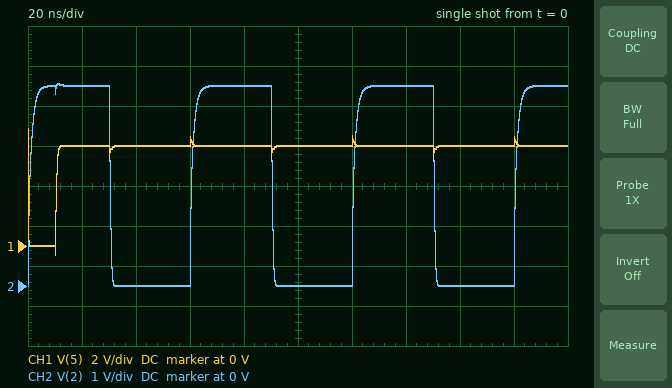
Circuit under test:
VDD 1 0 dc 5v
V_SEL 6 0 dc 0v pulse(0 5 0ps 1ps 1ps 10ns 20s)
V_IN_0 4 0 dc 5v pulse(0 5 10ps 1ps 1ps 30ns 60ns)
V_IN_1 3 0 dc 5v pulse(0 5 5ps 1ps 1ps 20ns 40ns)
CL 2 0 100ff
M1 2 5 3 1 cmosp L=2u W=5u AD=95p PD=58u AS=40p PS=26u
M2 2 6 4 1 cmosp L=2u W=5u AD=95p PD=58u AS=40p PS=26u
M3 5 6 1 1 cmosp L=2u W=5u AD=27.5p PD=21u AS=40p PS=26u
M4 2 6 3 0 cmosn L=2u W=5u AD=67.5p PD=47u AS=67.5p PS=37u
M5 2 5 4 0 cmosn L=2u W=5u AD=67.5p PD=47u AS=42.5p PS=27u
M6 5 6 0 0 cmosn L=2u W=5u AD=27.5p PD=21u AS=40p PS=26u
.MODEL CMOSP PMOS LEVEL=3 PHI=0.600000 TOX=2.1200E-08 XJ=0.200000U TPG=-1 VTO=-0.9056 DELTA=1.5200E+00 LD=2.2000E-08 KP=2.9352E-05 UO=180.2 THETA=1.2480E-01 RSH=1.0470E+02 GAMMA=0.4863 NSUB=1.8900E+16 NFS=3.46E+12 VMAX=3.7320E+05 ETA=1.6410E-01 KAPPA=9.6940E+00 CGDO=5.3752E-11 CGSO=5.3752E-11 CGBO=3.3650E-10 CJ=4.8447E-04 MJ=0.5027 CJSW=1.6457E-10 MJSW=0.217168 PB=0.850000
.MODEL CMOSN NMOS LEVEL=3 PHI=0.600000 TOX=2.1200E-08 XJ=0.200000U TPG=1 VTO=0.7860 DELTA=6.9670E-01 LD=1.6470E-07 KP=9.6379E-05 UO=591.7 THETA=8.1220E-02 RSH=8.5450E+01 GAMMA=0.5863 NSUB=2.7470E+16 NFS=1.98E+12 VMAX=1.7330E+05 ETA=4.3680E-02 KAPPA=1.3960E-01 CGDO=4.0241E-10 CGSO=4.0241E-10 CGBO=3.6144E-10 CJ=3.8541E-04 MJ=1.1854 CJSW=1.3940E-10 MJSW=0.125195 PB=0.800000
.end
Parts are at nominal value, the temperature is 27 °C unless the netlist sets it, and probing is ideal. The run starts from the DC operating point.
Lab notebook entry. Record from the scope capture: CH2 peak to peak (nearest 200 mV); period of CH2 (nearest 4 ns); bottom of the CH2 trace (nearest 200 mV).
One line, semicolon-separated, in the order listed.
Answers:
5.0 V; 60 ns; 0 V
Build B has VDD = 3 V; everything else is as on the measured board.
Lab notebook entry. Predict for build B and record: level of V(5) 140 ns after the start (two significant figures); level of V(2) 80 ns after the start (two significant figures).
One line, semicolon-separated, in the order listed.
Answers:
3.0 V; 3.5 V
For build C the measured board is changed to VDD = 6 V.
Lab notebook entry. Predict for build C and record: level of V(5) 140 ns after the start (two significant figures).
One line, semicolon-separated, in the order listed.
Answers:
6.0 V
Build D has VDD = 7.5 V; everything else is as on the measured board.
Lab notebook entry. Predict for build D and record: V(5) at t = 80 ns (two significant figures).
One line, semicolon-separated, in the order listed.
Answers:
7.5 V
